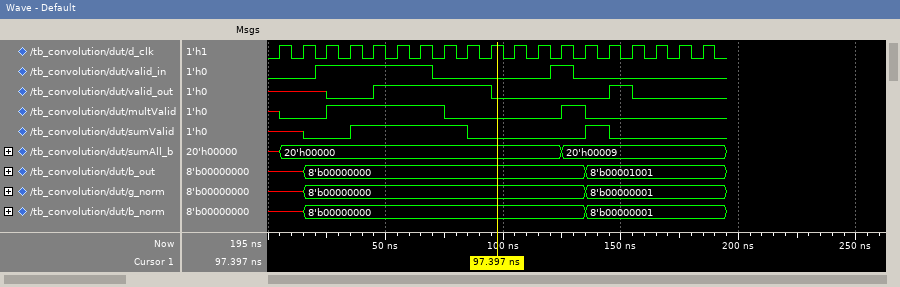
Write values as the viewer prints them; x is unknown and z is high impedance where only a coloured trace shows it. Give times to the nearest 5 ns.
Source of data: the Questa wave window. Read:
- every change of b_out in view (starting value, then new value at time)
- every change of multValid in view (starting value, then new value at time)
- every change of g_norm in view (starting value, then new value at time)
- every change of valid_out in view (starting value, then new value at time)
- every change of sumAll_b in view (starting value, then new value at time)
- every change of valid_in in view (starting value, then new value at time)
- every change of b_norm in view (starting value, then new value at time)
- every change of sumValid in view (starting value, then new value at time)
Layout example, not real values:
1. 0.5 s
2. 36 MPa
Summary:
1. x, 8'b00000000 at 15 ns, 8'b00001001 at 135 ns
2. x, 0 at 5 ns, 1 at 25 ns, 0 at 75 ns, 1 at 125 ns, 0 at 135 ns
3. x, 8'b00000000 at 15 ns, 8'b00000001 at 135 ns
4. x, 0 at 25 ns, 1 at 45 ns, 0 at 95 ns, 1 at 145 ns, 0 at 155 ns
5. x, 20'h00000 at 5 ns, 20'h00009 at 125 ns
6. 0, 1 at 20 ns, 0 at 70 ns, 1 at 120 ns, 0 at 130 ns
7. x, 8'b00000000 at 15 ns, 8'b00000001 at 135 ns
8. x, 0 at 15 ns, 1 at 35 ns, 0 at 85 ns, 1 at 135 ns, 0 at 145 ns
